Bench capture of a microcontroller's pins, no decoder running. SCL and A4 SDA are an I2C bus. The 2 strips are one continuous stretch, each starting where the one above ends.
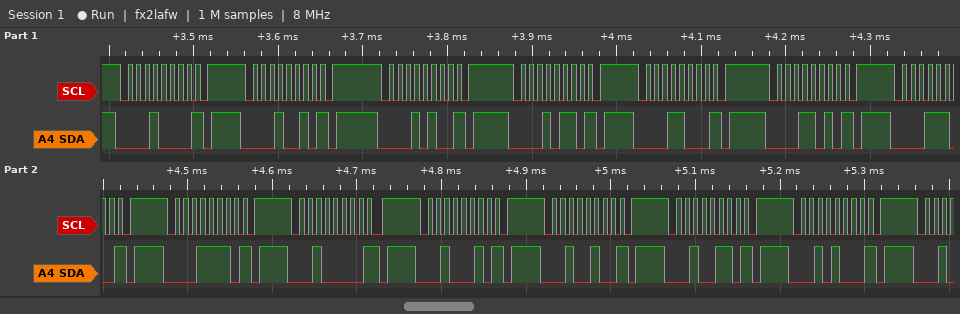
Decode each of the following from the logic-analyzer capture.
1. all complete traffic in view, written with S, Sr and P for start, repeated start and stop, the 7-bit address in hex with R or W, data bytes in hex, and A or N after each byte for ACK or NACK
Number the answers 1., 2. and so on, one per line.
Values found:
1. S 08W N P S 09W N P S 0AW N P S 0BW N P S 0CW N P S 0DW N P S 0EW N P S 0FW N P S 10W N P S 11W N P S 12W N P S 13W N P S 14W N P
